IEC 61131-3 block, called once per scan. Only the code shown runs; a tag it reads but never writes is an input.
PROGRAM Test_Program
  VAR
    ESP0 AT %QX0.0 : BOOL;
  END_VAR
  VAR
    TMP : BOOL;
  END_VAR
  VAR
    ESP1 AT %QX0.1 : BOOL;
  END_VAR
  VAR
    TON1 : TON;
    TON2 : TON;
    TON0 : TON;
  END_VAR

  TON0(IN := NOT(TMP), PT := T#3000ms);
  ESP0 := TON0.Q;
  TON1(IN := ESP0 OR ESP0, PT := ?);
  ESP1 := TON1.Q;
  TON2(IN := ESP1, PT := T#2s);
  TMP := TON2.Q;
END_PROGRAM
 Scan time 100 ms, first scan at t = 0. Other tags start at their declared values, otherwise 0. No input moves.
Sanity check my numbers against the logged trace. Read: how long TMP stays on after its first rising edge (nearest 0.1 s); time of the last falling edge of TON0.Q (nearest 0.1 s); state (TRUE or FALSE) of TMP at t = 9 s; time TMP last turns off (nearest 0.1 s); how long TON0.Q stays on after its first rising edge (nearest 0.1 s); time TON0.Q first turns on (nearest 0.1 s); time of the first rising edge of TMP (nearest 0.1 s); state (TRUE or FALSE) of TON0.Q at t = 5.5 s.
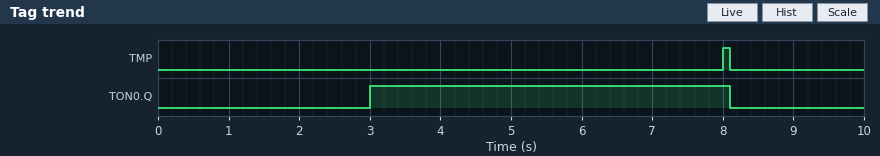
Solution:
0.1 s
8.1 s
FALSE
8.1 s
5.1 s
3.0 s
8.0 s
TRUE
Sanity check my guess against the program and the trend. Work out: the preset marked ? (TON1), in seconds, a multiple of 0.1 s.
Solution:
3.0 s
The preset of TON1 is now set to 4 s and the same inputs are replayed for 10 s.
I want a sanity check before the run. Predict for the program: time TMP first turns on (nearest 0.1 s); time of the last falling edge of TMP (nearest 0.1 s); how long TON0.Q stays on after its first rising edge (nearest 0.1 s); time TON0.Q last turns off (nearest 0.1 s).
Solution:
9.0 s
9.1 s
6.1 s
9.1 s
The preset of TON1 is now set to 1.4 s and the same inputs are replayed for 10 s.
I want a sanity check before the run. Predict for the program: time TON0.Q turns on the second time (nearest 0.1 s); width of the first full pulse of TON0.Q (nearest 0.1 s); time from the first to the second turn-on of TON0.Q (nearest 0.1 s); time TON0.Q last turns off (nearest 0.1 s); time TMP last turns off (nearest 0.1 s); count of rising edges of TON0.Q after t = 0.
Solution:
9.6 s
3.5 s
6.6 s
6.5 s
6.5 s
2
